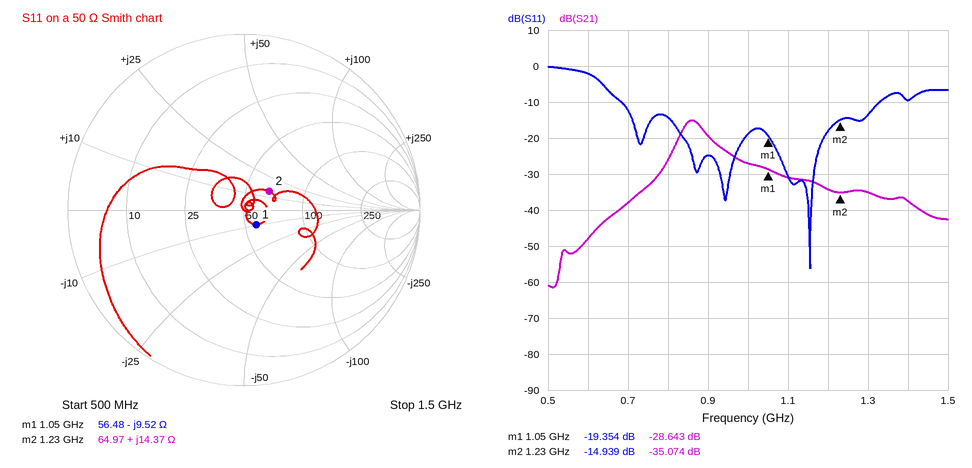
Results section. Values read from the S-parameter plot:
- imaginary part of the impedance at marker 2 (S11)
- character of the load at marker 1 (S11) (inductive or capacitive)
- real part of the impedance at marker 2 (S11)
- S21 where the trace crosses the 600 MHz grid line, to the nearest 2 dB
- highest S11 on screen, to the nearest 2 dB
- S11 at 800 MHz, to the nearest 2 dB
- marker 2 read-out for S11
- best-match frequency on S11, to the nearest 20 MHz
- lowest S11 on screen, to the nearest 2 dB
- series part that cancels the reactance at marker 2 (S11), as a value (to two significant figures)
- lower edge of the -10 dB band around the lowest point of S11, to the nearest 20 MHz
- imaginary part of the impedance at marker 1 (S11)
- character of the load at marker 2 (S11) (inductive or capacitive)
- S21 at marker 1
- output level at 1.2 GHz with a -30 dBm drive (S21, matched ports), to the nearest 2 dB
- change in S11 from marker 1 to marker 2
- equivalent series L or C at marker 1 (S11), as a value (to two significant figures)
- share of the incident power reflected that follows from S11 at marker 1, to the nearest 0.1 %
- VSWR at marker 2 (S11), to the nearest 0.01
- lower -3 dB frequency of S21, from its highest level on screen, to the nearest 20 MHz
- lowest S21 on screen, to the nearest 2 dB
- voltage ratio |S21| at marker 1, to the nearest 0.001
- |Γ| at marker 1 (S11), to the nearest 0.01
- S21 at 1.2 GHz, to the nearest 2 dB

+14.37 Ω
capacitive
64.97 Ω
-48 dB
0 dB
-14 dB
-14.939 dB
1.16 GHz
-56 dB
9.0 pF
680 MHz
-9.52 Ω
inductive
-28.643 dB
-64 dBm
4.415 dB
16 pF
1.2 %
1.44
840 MHz
-62 dB
0.037
0.11
-34 dB
